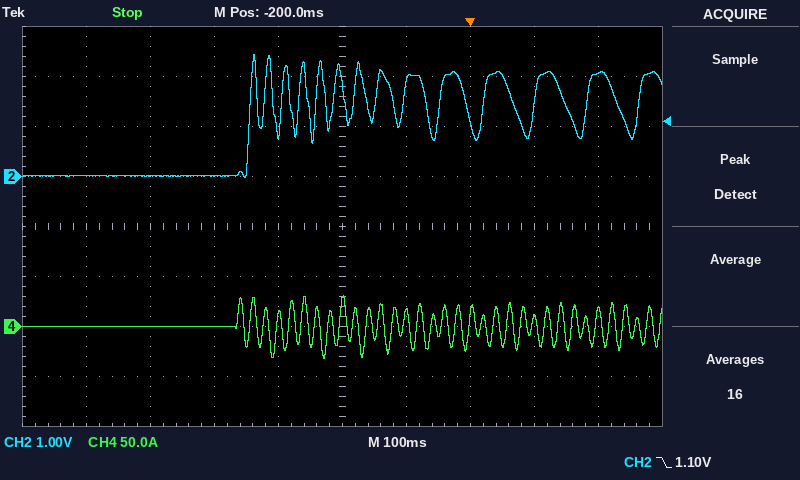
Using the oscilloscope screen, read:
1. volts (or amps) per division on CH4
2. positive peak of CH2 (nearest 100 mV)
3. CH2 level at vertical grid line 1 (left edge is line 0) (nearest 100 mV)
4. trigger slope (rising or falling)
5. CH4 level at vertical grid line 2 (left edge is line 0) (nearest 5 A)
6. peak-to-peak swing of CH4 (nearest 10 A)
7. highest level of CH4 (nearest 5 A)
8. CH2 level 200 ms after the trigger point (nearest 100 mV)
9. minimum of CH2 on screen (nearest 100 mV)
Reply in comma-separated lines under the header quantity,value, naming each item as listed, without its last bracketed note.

quantity,value
volts (or amps) per division on CH4,50 A
positive peak of CH2,2.4 V
CH2 level at vertical grid line 1 (left edge is line 0),0.0 V
trigger slope,falling
CH4 level at vertical grid line 2 (left edge is line 0),0 A
peak-to-peak swing of CH4,60 A
highest level of CH4,30 A
CH2 level 200 ms after the trigger point,2.1 V
minimum of CH2 on screen,0.0 V
